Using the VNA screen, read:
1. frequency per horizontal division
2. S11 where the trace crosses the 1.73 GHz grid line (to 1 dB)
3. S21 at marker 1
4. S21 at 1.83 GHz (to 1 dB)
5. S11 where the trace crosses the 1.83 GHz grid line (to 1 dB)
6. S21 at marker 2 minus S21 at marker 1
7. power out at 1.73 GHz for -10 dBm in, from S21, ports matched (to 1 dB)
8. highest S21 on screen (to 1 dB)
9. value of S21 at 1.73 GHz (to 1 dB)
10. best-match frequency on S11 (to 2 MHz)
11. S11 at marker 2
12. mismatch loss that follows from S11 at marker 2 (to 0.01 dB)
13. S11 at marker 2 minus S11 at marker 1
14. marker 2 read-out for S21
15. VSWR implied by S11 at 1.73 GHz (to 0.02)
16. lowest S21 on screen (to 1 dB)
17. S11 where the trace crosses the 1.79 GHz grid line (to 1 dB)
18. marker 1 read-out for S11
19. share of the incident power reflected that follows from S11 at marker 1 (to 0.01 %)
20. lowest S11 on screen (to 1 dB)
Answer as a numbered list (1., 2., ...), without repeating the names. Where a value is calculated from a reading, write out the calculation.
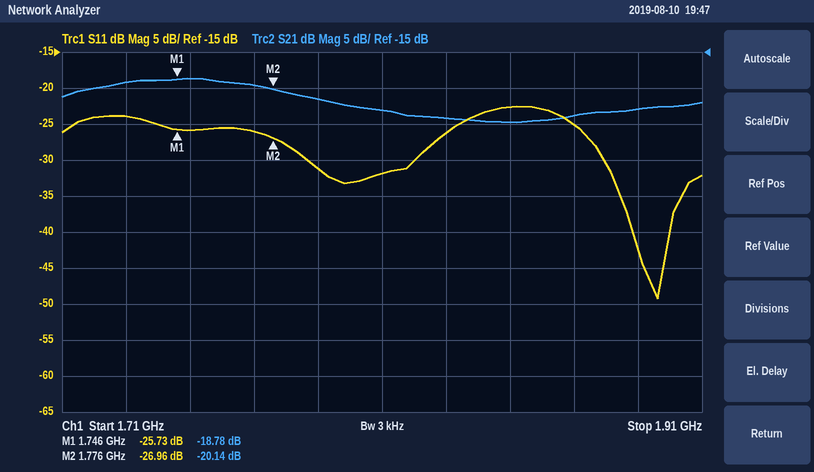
1. 20 MHz
2. -24 dB
3. -18.78 dB
4. -24 dB
5. -26 dB
6. -20.14 − (-18.78) = -1.36 dB
7. -10 dBm + (-19 dB) = -29 dBm
8. -19 dB
9. -19 dB
10. 1.896 GHz
11. -26.96 dB
12. −10 log10(1 − 10^(-26.96/10)) ≈ 0.01 dB
13. -26.96 − (-25.73) = -1.23 dB
14. -20.14 dB
15. |Γ| = 10^(-24/20) = 0.0631; VSWR = (1 + 0.0631)/(1 − 0.0631) ≈ 1.13, so 1.14 to the nearest 0.02
16. -25 dB
17. -31 dB
18. -25.73 dB
19. 10^(-25.73/10) ≈ 0.27 %
20. -49 dB
